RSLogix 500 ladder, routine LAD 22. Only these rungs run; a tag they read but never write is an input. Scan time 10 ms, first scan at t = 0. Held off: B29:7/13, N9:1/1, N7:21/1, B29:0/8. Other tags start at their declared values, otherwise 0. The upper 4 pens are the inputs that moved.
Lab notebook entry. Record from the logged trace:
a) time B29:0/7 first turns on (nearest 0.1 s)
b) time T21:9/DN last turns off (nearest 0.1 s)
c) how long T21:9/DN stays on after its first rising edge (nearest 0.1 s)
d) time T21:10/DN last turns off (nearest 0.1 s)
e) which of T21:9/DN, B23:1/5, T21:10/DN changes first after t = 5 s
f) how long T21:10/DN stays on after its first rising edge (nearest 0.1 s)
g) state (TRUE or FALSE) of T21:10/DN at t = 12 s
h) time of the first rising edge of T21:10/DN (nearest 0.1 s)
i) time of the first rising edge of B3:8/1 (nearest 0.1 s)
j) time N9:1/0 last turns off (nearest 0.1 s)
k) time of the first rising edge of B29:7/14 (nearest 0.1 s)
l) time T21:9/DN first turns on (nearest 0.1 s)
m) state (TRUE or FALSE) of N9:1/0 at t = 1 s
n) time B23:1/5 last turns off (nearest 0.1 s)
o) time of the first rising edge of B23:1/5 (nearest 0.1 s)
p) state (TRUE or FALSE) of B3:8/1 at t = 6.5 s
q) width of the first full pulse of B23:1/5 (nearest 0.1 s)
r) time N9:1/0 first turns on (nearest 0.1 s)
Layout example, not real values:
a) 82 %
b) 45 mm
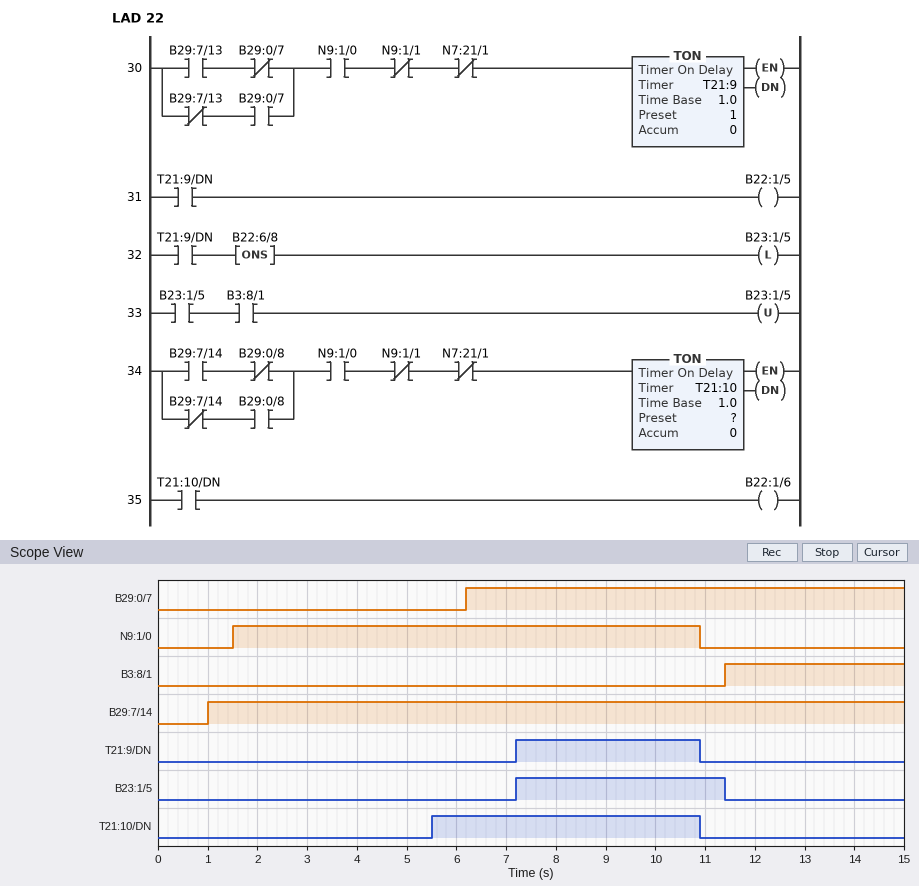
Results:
a) 6.2 s
b) 10.9 s
c) 3.7 s
d) 10.9 s
e) T21:10/DN
f) 5.4 s
g) FALSE
h) 5.5 s
i) 11.4 s
j) 10.9 s
k) 1.0 s
l) 7.2 s
m) FALSE
n) 11.4 s
o) 7.2 s
p) FALSE
q) 4.2 s
r) 1.5 s
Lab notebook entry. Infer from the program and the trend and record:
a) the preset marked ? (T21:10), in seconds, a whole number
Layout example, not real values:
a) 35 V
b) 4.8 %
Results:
a) 4 s
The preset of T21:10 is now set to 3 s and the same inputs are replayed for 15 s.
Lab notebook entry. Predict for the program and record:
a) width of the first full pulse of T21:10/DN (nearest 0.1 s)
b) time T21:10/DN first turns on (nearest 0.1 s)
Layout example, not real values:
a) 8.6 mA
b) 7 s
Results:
a) 6.4 s
b) 4.5 s
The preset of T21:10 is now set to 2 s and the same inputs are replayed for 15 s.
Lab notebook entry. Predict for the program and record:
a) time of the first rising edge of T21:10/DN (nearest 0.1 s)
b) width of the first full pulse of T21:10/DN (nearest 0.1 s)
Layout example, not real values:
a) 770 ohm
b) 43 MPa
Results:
a) 3.5 s
b) 7.4 s
